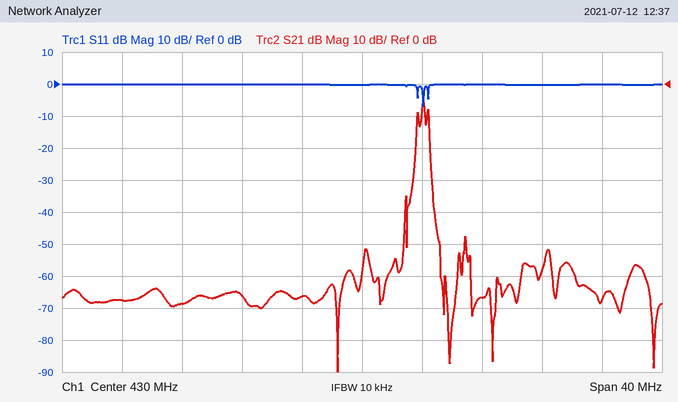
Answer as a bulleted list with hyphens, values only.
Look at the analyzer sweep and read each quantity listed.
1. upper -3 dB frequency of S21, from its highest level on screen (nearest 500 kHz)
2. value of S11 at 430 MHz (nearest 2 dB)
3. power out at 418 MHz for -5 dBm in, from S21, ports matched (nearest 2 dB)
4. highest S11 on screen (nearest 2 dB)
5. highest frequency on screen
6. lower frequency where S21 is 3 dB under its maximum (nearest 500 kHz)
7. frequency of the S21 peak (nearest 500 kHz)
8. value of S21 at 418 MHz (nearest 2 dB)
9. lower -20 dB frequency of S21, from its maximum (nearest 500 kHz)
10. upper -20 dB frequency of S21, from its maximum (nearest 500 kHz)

- 434.0 MHz
- 0 dB
- -74 dBm
- 0 dB
- 450 MHz
- 434.0 MHz
- 434.0 MHz
- -68 dB
- 433.5 MHz
- 434.5 MHz
